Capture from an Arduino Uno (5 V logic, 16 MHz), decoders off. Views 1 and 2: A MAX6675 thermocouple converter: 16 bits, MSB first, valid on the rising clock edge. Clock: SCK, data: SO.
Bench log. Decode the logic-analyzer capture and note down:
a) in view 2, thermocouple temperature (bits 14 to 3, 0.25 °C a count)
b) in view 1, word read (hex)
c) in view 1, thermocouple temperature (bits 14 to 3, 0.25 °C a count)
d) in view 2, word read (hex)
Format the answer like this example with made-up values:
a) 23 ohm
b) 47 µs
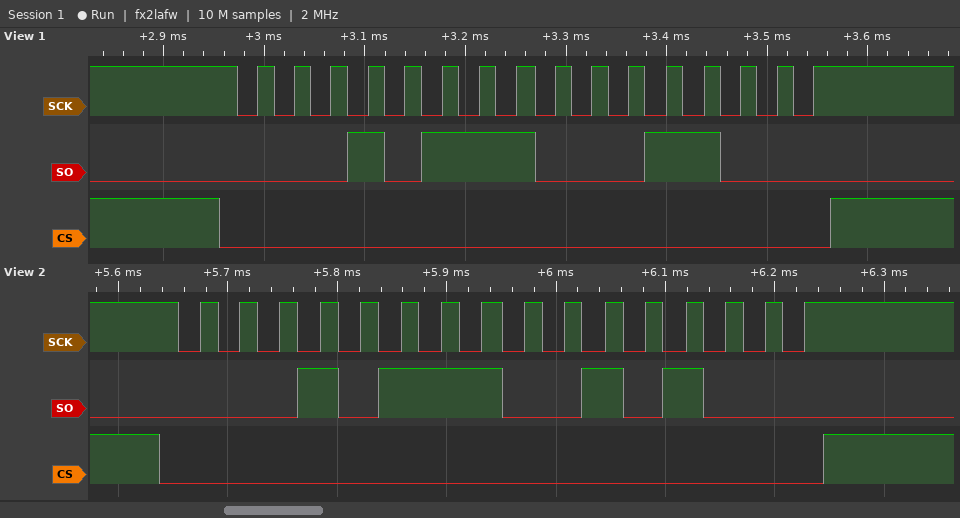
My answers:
a) 185.25 °C
b) 0x1718
c) 184.75 °C
d) 0x1728
